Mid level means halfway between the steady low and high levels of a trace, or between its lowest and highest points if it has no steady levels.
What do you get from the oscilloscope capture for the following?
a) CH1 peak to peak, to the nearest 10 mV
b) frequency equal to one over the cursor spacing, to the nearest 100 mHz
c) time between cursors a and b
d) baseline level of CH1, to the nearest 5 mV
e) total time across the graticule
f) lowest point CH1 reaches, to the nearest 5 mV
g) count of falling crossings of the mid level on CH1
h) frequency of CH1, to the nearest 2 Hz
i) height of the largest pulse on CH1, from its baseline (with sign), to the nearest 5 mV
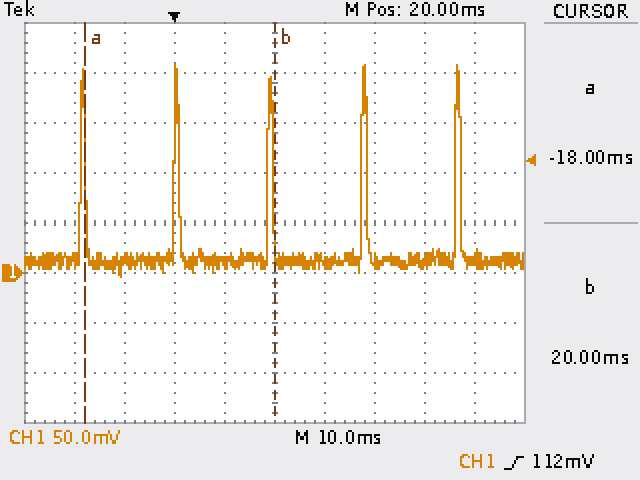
210 mV
26.3 Hz
38 ms
10 mV
100 ms
-5 mV
5
54 Hz
+195 mV
